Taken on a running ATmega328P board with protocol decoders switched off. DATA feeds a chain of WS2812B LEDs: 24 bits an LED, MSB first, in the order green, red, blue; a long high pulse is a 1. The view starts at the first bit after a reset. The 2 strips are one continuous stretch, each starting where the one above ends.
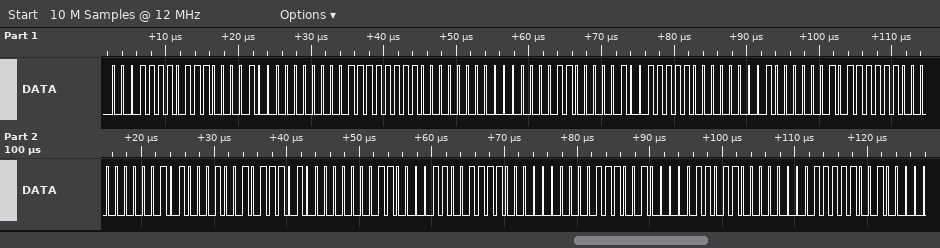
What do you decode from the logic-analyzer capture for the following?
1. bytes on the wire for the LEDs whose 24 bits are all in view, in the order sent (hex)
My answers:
1E E1 00 3F C0 00 60 9F 00 81 7E 00 A2 5D 00 C3 3C 00 E4 1B 00
